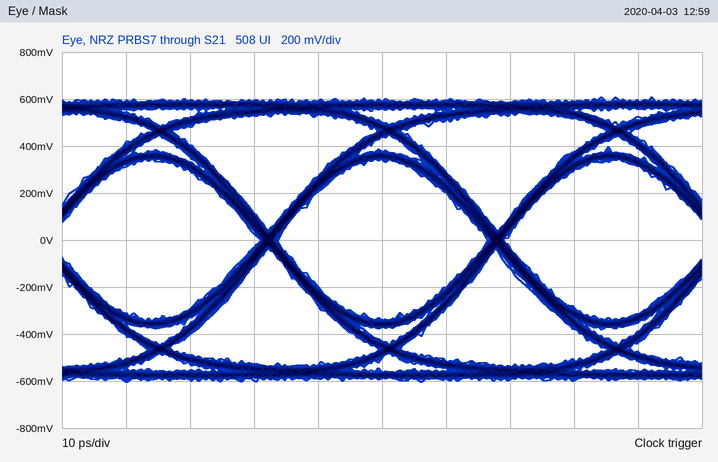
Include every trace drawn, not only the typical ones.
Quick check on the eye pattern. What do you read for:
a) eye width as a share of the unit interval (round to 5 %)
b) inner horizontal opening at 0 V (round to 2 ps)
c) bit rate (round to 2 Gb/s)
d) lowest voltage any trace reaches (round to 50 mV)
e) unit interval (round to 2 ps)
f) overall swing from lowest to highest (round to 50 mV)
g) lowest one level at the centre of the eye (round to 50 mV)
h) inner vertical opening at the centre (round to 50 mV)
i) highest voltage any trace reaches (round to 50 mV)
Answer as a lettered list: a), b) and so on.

a) 90 %
b) 32 ps
c) 28 Gb/s
d) -600 mV
e) 36 ps
f) 1.20 V
g) 350 mV
h) 700 mV
i) 600 mV
